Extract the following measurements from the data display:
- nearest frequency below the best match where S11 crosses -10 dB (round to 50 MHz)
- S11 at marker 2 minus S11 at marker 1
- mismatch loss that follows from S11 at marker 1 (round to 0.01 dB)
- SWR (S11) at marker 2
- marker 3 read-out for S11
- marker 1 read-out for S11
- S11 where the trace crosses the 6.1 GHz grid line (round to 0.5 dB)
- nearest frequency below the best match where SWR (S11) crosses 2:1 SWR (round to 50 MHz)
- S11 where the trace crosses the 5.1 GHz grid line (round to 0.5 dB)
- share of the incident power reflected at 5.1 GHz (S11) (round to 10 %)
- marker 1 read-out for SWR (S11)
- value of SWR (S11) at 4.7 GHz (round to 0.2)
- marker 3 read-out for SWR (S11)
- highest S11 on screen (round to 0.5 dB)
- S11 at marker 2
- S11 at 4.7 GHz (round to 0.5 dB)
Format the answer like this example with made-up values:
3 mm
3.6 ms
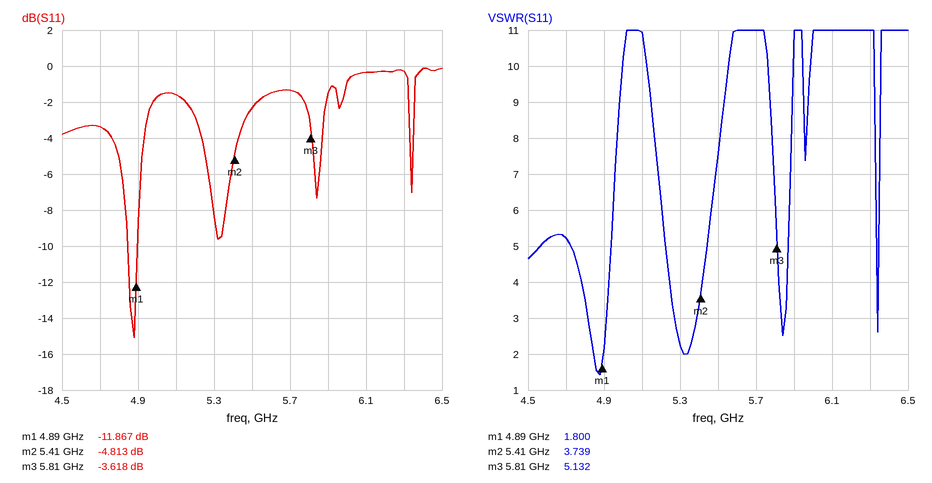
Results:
4.85 GHz
7.054 dB
0.29 dB
3.739
-3.618 dB
-11.867 dB
-0.5 dB
4.85 GHz
-1.5 dB
70 %
1.800
5.2
5.132
0.0 dB
-4.813 dB
-3.5 dB
